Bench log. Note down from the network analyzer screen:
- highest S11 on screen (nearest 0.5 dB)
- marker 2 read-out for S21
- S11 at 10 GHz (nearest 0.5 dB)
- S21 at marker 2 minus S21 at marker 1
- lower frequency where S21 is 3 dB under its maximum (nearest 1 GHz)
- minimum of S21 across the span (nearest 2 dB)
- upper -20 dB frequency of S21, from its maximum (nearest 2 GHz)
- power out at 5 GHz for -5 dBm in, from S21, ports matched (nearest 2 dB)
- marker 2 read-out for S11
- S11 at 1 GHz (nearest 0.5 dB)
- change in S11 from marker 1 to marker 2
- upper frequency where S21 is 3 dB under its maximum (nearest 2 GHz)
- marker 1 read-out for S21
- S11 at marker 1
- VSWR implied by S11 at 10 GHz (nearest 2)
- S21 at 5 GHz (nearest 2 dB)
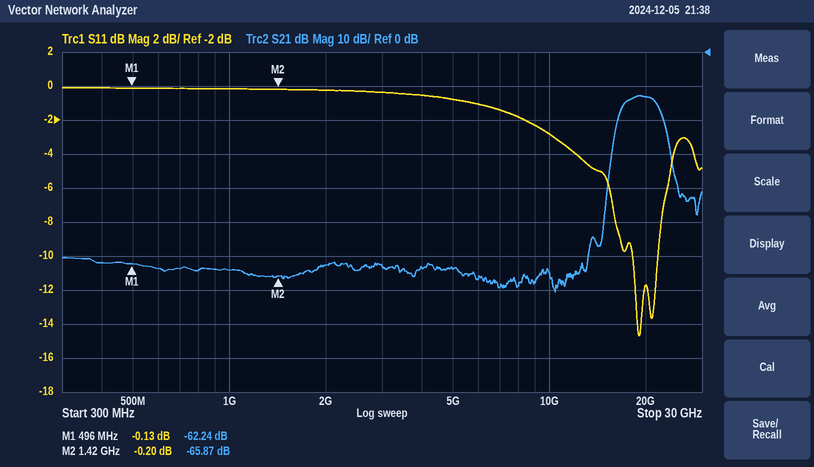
0.0 dB
-65.87 dB
-3.0 dB
-3.63 dB
17 GHz
-70 dB
24 GHz
-68 dBm
-0.20 dB
0.0 dB
-0.07 dB
22 GHz
-62.24 dB
-0.13 dB
6
-64 dB
